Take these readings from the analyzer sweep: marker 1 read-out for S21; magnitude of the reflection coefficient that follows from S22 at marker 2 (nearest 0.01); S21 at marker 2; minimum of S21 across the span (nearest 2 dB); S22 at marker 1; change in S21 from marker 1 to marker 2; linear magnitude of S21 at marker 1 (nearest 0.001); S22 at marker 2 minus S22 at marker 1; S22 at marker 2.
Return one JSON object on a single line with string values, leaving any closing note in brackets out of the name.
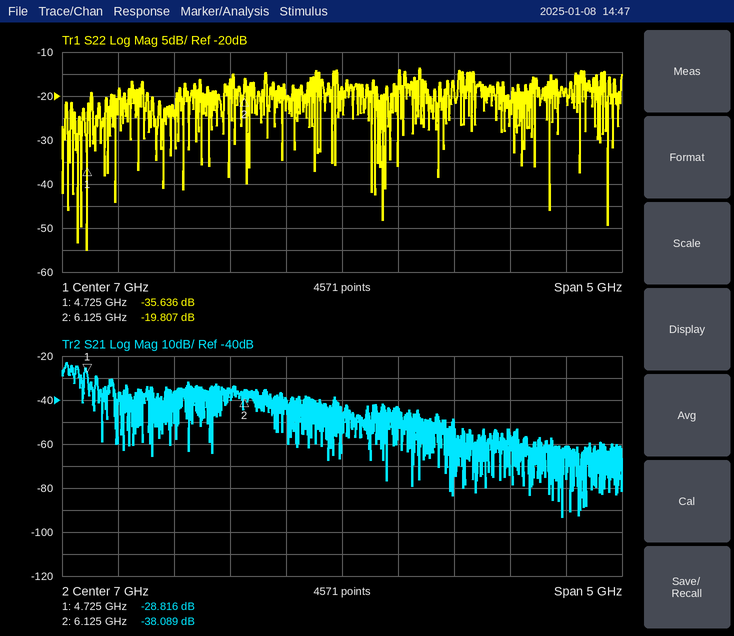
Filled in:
{"marker 1 read-out for S21": "-28.816 dB", "magnitude of the reflection coefficient that follows from S22 at marker 2": "0.10", "S21 at marker 2": "-38.089 dB", "minimum of S21 across the span": "-94 dB", "S22 at marker 1": "-35.636 dB", "change in S21 from marker 1 to marker 2": "-9.273 dB", "linear magnitude of S21 at marker 1": "0.036", "S22 at marker 2 minus S22 at marker 1": "15.829 dB", "S22 at marker 2": "-19.807 dB"}
